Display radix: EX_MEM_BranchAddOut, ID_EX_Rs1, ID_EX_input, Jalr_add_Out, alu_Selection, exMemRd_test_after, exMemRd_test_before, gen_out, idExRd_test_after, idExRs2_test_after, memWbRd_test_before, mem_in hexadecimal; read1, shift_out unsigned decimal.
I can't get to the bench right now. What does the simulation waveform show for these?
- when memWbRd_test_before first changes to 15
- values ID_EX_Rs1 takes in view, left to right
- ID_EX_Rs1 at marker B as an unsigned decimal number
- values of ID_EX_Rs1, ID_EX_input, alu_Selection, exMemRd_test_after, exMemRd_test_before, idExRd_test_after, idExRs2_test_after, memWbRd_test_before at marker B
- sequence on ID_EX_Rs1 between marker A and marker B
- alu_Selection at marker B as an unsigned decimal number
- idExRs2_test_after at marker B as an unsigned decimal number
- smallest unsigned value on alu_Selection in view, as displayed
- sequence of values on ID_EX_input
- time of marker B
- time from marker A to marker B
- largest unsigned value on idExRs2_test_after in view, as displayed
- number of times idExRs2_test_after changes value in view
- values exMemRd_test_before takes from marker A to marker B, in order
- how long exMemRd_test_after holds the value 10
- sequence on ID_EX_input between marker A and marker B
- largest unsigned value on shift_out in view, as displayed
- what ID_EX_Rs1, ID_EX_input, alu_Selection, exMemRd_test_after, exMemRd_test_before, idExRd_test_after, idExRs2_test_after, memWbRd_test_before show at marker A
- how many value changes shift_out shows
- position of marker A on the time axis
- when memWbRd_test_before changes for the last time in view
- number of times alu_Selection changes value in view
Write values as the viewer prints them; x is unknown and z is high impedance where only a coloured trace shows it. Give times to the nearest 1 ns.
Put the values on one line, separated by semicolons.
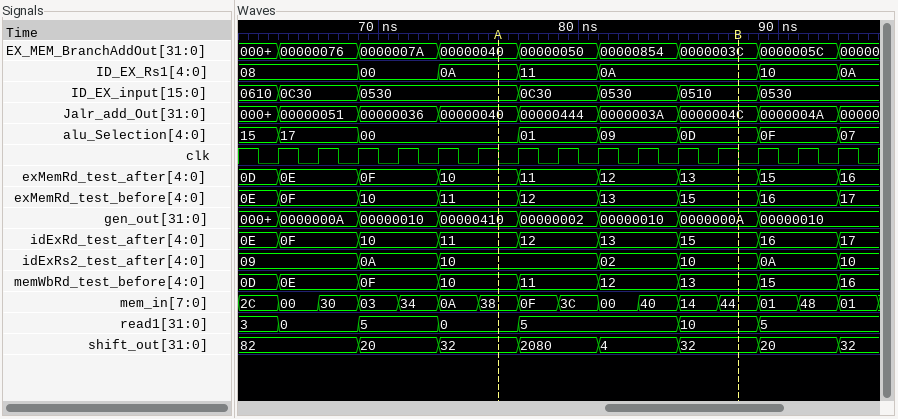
89 ns; 08, 00, 0A, 11, 0A, 10, 0A; 10; ID_EX_Rs1=0A, ID_EX_input=0510, alu_Selection=0D, exMemRd_test_after=13, exMemRd_test_before=15, idExRd_test_after=15, idExRs2_test_after=10, memWbRd_test_before=13; 0A, 11, 0A; 13; 16; 00; 0610, 0C30, 0530, 0C30, 0530, 0510, 0530; 88 ns; 12 ns; 10; 6; 11, 12, 13, 15; 4 ns; 0530, 0C30, 0530, 0510; 2080; ID_EX_Rs1=0A, ID_EX_input=0530, alu_Selection=00, exMemRd_test_after=10, exMemRd_test_before=11, idExRd_test_after=11, idExRs2_test_after=10, memWbRd_test_before=10; 7; 76 ns; 93 ns; 7
